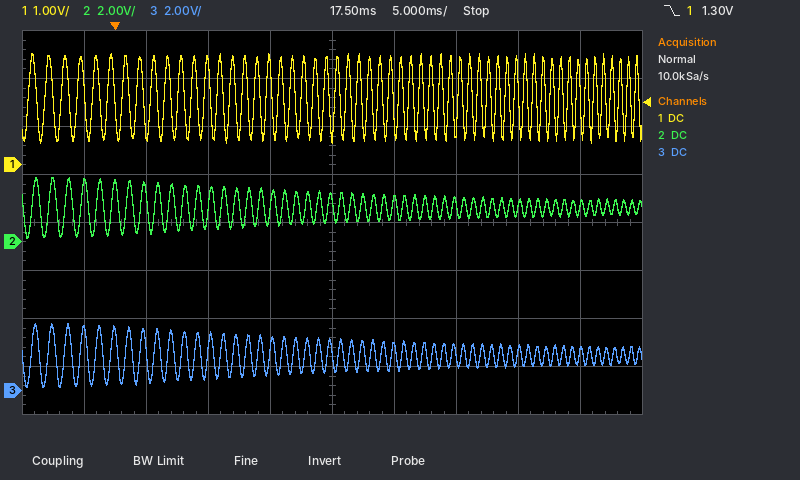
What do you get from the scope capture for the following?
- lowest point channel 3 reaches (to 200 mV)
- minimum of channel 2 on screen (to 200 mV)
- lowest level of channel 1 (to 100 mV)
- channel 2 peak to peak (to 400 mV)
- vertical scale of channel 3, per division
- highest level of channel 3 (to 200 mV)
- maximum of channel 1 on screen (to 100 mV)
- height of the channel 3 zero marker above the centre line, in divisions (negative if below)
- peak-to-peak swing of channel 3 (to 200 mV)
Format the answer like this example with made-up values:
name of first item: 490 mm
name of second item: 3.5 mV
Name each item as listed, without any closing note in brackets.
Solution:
lowest point channel 3 reaches: 200 mV
minimum of channel 2 on screen: 200 mV
lowest level of channel 1: 500 mV
channel 2 peak to peak: 2.4 V
vertical scale of channel 3, per division: 2 V
highest level of channel 3: 2.8 V
maximum of channel 1 on screen: 2.3 V
height of the channel 3 zero marker above the centre line, in divisions: -3.5 div
peak-to-peak swing of channel 3: 2.6 V
